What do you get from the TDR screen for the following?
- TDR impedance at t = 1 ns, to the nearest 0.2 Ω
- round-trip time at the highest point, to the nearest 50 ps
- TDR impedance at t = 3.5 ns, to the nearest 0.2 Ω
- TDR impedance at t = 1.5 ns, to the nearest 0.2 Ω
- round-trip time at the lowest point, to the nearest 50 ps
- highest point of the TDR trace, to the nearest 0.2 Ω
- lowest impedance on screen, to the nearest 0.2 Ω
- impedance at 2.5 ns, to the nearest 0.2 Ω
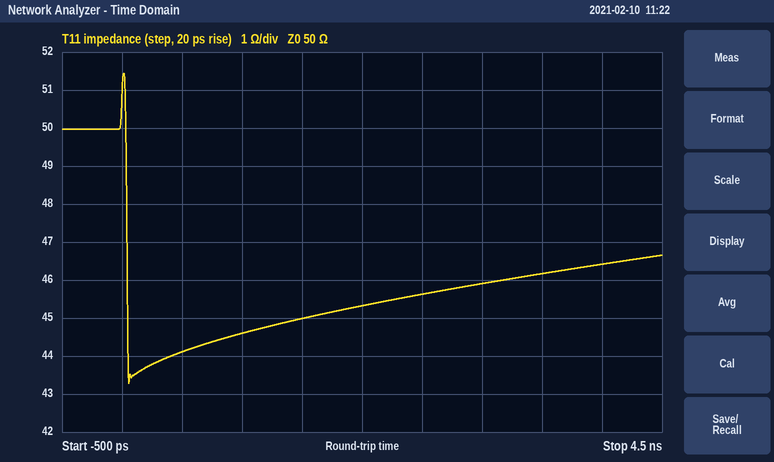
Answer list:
44.6 Ω
0 ps
46.2 Ω
45.0 Ω
50 ps
51.4 Ω
43.2 Ω
45.6 Ω
